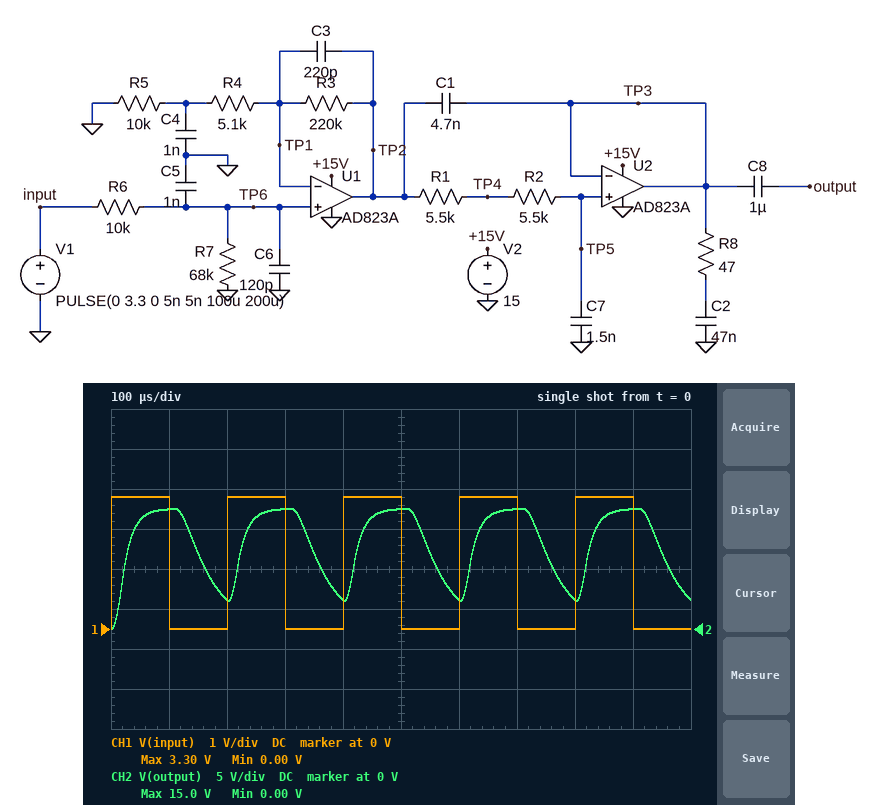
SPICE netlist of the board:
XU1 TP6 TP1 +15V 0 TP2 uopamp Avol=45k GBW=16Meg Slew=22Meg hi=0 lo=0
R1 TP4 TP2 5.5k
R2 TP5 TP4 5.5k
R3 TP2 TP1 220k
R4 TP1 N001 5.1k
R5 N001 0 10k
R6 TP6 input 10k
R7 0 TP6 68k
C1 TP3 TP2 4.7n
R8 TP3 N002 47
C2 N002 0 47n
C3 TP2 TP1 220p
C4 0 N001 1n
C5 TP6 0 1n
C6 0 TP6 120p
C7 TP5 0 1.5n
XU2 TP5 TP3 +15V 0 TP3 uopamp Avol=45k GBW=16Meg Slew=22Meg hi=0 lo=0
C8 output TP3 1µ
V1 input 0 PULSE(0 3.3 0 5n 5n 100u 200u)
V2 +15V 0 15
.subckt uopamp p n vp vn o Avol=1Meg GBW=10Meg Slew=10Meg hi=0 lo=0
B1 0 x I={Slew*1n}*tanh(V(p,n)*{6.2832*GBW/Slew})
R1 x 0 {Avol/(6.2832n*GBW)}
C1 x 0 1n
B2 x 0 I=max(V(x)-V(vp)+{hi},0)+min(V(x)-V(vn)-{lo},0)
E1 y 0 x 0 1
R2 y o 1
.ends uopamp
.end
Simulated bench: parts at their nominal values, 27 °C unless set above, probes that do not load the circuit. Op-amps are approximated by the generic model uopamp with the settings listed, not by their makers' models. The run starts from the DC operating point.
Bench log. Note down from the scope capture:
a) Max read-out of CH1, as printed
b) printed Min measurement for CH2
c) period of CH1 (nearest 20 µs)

3.30 V
0.00 V
200 µs
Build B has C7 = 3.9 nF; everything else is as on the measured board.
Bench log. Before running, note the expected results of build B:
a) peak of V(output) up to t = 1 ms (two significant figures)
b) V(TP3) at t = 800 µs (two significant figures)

14 V
6.2 V
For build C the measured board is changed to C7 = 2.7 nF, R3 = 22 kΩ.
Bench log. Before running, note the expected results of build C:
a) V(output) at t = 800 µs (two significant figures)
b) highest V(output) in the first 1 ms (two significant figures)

330 mV
6.7 V
